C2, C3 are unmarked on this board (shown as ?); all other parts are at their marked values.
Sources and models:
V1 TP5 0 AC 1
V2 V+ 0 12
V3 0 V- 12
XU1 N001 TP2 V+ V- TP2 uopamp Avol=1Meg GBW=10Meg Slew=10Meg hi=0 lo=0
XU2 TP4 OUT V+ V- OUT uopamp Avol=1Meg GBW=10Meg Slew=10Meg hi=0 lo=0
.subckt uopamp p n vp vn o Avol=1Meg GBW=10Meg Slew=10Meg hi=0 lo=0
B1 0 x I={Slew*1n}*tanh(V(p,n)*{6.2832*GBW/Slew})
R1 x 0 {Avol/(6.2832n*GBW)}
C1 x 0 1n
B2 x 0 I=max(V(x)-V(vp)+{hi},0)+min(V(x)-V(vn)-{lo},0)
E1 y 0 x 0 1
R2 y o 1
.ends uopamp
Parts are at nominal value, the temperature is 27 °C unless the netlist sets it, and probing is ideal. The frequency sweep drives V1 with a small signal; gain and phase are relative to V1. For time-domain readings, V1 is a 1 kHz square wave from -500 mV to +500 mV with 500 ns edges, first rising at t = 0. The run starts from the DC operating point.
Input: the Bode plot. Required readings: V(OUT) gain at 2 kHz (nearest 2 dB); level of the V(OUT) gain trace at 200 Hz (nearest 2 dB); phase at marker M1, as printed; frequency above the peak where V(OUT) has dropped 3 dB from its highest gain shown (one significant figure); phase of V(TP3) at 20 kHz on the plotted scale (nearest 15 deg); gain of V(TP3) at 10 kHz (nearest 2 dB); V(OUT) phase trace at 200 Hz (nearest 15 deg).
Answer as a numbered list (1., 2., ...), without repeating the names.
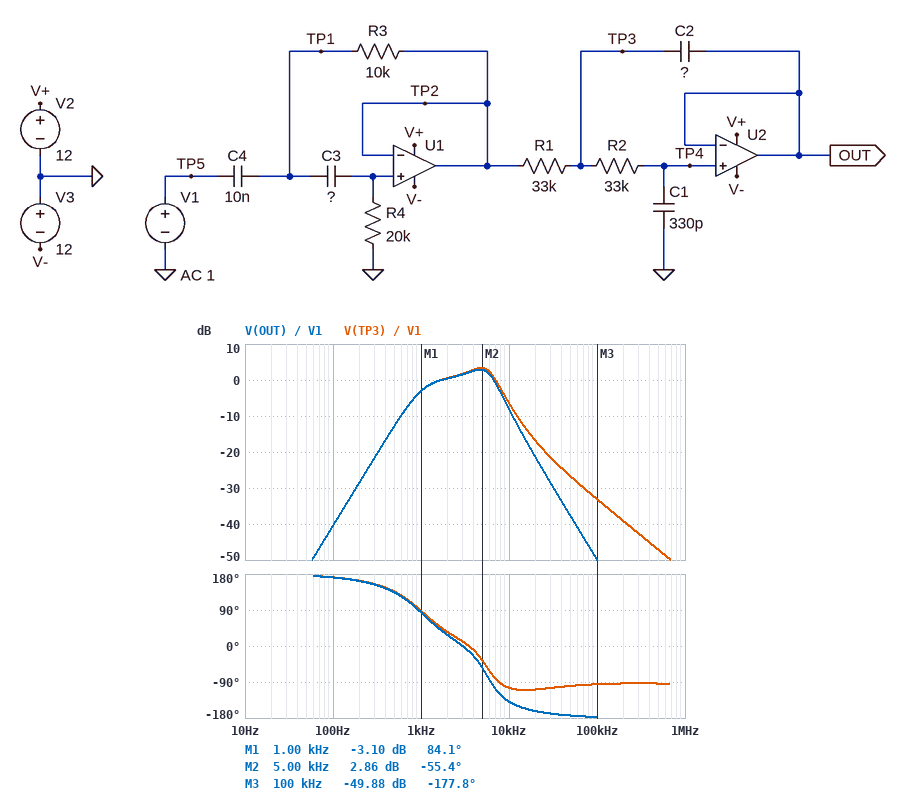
1. 0 dB
2. -28 dB
3. 84.1 deg
4. 7 kHz
5. -105 deg
6. -6 dB
7. 165 deg
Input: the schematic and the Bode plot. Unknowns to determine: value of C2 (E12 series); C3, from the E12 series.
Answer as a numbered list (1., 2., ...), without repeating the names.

1. 2.2 nF
2. 12 nF
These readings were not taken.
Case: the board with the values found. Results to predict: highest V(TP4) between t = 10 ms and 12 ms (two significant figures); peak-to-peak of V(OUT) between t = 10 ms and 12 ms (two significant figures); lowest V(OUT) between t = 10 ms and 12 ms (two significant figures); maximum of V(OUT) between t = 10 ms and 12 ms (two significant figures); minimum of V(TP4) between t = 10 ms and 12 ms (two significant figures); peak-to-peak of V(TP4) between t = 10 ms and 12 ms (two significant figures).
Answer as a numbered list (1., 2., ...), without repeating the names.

1. 950 mV
2. 1.9 V
3. -950 mV
4. 950 mV
5. -950 mV
6. 1.9 V
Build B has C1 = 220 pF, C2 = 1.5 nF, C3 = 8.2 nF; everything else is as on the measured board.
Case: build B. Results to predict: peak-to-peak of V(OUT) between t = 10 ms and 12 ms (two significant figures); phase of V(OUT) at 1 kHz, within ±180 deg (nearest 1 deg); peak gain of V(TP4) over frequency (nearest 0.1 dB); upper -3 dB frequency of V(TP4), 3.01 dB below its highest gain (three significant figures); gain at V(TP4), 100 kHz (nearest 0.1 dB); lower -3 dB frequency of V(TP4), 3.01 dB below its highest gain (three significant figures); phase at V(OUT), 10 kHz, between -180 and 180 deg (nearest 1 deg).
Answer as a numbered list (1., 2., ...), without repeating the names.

1. 1.9 V
2. 102 deg
3. 3.0 dB
4. 9.98 kHz
5. -43.0 dB
6. 2.22 kHz
7. -105 deg
